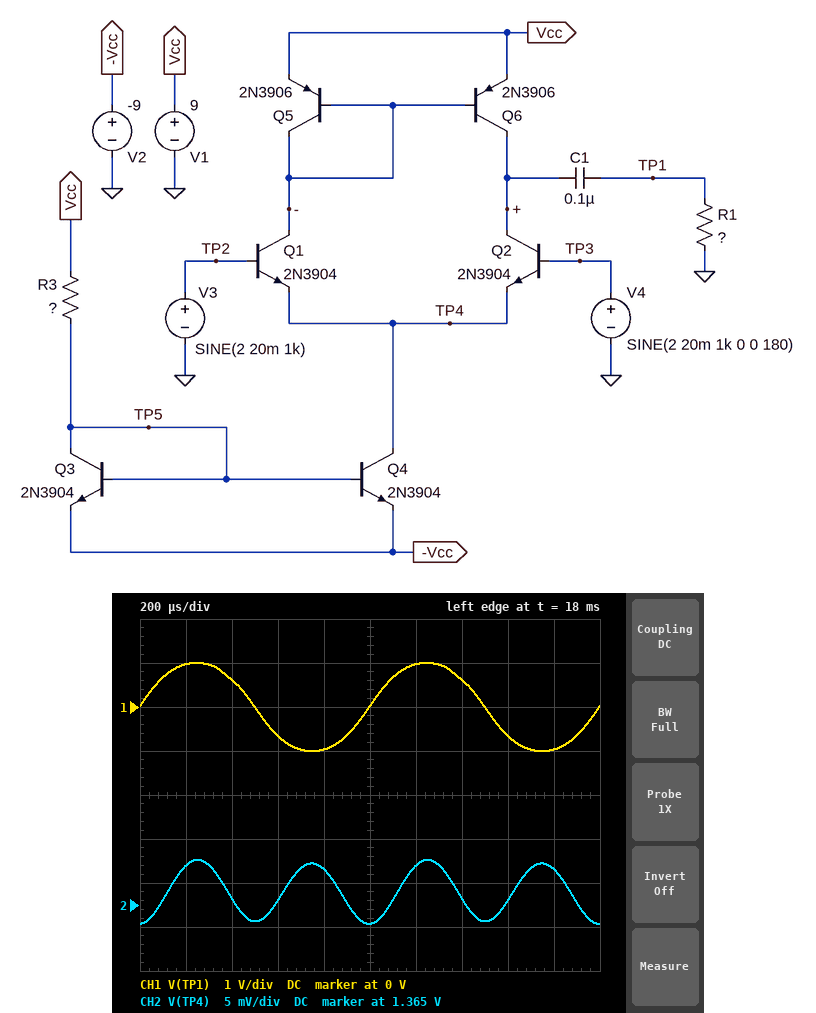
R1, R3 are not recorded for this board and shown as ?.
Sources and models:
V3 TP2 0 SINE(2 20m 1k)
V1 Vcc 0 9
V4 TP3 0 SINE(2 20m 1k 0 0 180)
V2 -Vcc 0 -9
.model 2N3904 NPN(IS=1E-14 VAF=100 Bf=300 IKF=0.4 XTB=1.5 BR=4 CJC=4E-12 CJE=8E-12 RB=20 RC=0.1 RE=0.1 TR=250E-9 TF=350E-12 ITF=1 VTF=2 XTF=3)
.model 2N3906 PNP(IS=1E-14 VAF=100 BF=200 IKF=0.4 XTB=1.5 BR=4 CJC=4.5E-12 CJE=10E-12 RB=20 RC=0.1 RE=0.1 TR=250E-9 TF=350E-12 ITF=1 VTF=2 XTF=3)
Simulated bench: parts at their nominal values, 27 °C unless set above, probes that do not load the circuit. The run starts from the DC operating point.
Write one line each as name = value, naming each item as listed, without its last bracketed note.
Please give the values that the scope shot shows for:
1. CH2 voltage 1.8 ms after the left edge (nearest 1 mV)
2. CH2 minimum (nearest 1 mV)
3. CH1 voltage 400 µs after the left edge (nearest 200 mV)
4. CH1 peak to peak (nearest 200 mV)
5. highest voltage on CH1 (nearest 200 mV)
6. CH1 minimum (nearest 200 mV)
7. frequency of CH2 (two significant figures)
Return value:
CH2 voltage 1.8 ms after the left edge = 1.369 V
CH2 minimum = 1.363 V
CH1 voltage 400 µs after the left edge = 600 mV
CH1 peak to peak = 2.0 V
highest voltage on CH1 = 1.0 V
CH1 minimum = -1.0 V
frequency of CH2 = 2.0 kHz
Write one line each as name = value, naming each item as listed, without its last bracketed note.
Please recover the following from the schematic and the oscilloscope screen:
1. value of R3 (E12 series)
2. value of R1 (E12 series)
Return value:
value of R3 = 18 kΩ
value of R1 = 1.5 kΩ
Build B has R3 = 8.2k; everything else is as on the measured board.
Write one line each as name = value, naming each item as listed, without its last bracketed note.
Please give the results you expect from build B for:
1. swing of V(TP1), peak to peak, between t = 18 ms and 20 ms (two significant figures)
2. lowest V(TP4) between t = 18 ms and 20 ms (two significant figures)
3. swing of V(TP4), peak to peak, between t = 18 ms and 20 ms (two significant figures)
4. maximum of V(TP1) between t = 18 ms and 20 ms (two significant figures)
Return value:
swing of V(TP1), peak to peak, between t = 18 ms and 20 ms = 4.3 V
lowest V(TP4) between t = 18 ms and 20 ms = 1.3 V
swing of V(TP4), peak to peak, between t = 18 ms and 20 ms = 7.5 mV
maximum of V(TP1) between t = 18 ms and 20 ms = 2.2 V
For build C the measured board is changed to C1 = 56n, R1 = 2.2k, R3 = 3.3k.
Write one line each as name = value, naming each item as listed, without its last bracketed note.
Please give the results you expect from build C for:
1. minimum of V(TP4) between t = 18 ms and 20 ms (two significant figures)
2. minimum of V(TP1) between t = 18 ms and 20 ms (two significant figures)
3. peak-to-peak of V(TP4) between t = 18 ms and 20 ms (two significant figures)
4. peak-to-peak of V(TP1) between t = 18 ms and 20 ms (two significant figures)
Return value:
minimum of V(TP4) between t = 18 ms and 20 ms = 1.3 V
minimum of V(TP1) between t = 18 ms and 20 ms = -4.9 V
peak-to-peak of V(TP4) between t = 18 ms and 20 ms = 20 mV
peak-to-peak of V(TP1) between t = 18 ms and 20 ms = 9.8 V
